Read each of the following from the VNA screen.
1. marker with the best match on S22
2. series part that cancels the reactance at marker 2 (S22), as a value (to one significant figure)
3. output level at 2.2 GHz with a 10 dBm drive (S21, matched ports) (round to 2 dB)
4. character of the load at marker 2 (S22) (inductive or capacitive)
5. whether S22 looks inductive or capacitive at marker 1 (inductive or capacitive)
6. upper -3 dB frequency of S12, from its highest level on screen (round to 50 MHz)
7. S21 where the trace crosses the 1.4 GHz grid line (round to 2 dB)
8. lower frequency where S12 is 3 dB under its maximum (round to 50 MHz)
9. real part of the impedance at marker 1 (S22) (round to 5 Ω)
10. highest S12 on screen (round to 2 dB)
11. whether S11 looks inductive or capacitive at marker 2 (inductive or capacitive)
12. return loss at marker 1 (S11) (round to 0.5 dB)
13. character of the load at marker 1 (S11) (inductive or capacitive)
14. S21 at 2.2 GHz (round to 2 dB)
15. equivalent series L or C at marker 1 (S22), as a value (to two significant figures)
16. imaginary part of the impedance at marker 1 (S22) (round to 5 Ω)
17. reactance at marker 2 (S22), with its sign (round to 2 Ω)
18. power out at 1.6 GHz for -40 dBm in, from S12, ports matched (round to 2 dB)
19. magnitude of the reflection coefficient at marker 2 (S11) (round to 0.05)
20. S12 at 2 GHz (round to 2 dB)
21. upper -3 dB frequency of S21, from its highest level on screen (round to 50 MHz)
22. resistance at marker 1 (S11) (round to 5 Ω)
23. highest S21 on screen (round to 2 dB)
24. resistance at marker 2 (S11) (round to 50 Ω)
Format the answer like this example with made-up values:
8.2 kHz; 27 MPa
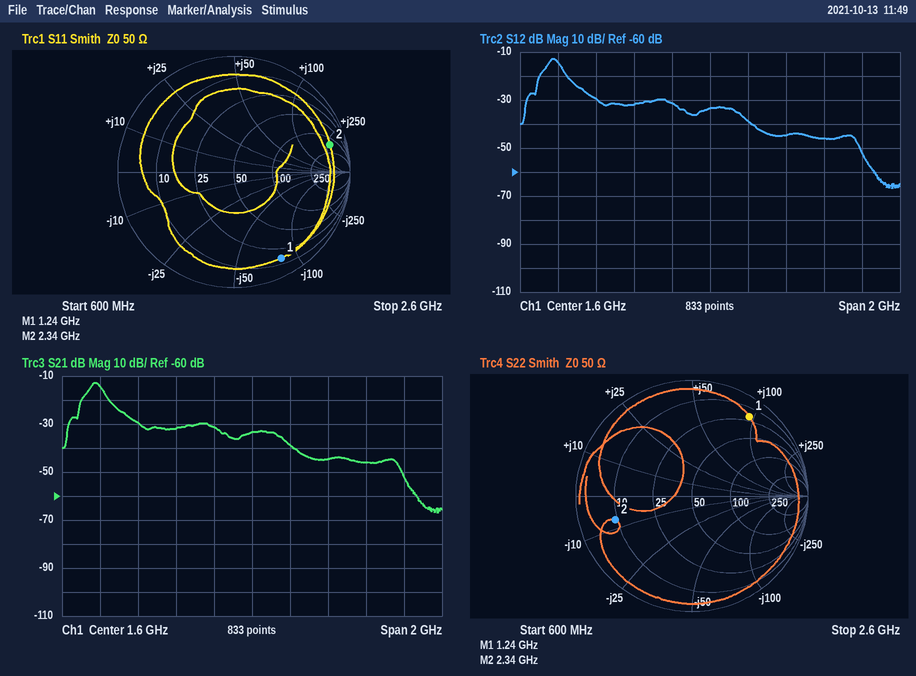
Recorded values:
marker 2; 500 pH; -36 dBm; capacitive; inductive; 800 MHz; -32 dB; 750 MHz; 20 Ω; -12 dB; inductive; 1.5 dB; capacitive; -46 dB; 12 nH; +95 Ω; -8 Ω; -74 dBm; 0.85; -44 dB; 800 MHz; 15 Ω; -12 dB; 150 Ω
